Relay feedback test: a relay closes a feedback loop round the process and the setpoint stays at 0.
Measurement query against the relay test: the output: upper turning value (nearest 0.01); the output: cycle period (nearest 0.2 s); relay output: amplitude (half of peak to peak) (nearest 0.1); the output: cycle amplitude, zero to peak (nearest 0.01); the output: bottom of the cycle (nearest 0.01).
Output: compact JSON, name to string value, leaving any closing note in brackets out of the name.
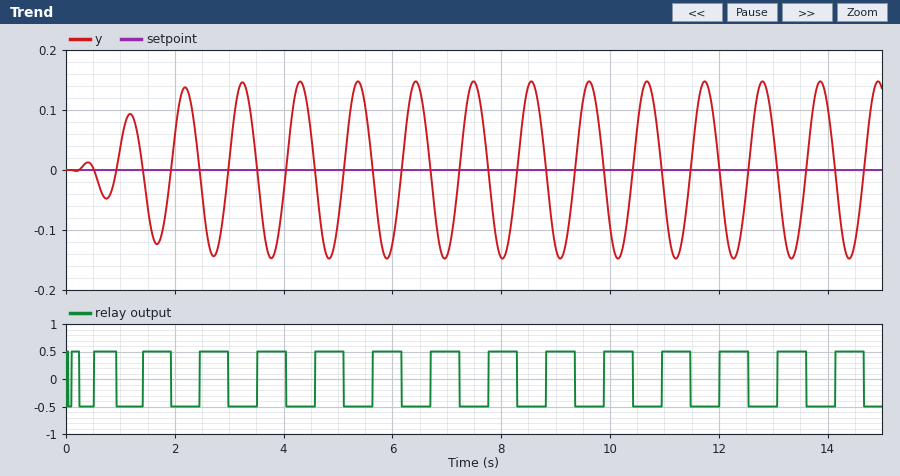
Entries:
{"the output: upper turning value": "0.15", "the output: cycle period": "1.0 s", "relay output: amplitude (half of peak to peak)": "0.5", "the output: cycle amplitude, zero to peak": "0.15", "the output: bottom of the cycle": "-0.15"}
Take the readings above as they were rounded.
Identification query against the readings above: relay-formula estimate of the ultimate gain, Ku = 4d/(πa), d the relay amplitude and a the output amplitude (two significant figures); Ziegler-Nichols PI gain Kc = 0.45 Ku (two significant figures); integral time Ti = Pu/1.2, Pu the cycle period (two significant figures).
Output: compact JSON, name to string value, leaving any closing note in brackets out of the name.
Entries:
{"relay-formula estimate of the ultimate gain, Ku = 4d/(πa), d the relay amplitude and a the output amplitude": "4.2", "Ziegler-Nichols PI gain Kc = 0.45 Ku": "1.9", "integral time Ti = Pu/1.2, Pu the cycle period": "0.83 s"}
